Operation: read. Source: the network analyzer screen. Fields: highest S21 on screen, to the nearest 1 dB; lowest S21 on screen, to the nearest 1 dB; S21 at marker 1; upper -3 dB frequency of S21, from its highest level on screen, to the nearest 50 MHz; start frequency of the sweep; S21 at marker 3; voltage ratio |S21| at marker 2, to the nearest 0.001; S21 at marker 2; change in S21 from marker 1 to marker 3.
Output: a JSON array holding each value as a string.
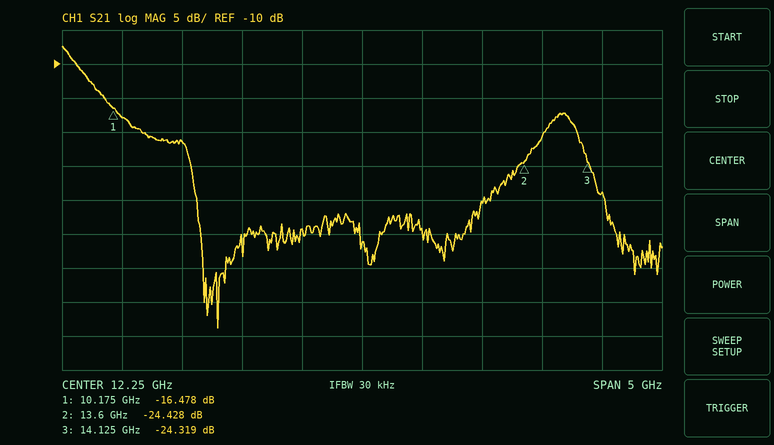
["-7 dB", "-49 dB", "-16.478 dB", "9.90 GHz", "9.75 GHz", "-24.319 dB", "0.060", "-24.428 dB", "-7.841 dB"]
